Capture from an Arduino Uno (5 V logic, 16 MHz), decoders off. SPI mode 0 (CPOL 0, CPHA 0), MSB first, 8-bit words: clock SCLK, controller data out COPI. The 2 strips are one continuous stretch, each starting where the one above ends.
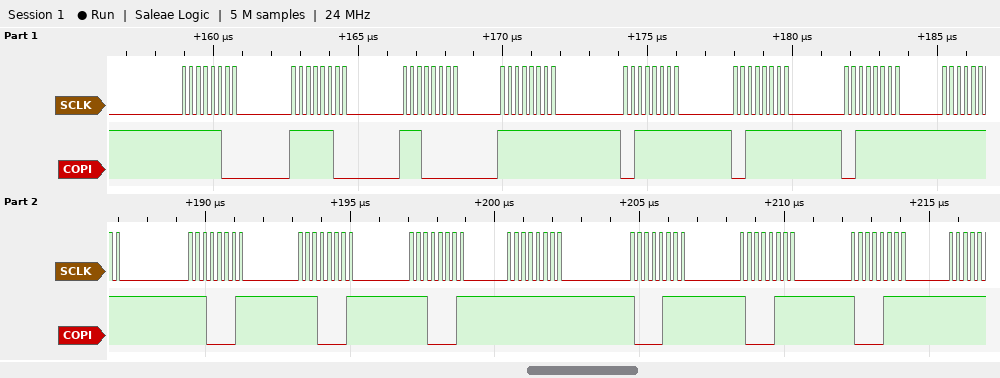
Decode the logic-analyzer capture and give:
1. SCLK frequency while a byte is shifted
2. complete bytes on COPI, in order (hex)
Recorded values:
4 MHz
0xFC 0xFC 0xE0 0xFF 0x3F 0x3F 0x3F 0xFF 0xE1 0xE1 0xE1 0xFF 0x87 0x87 0x87
